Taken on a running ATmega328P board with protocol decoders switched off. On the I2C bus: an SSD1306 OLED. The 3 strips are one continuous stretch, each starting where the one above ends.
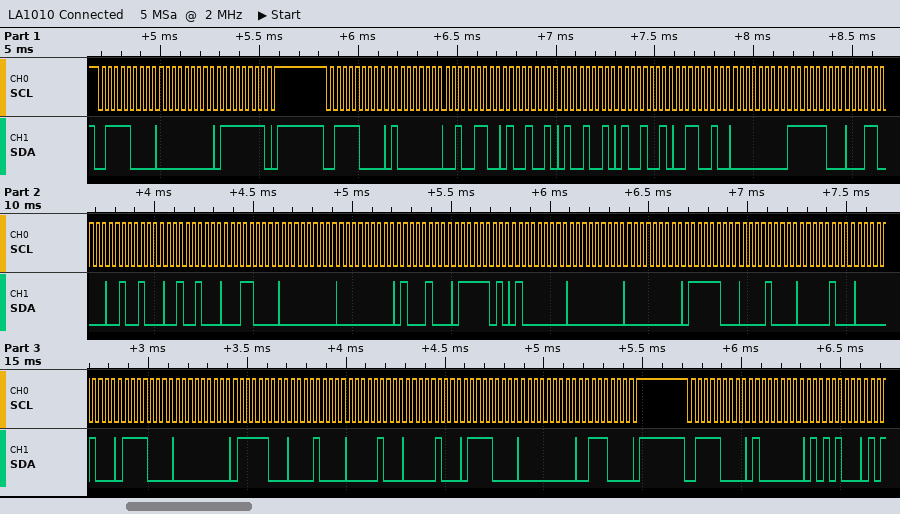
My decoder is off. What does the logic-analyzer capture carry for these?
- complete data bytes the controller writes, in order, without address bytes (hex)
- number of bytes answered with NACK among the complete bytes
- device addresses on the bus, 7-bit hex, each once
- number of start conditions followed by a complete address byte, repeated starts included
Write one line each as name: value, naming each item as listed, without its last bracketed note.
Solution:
complete data bytes the controller writes, in order, without address bytes: 00 7F 40 26 49 49 49 32 00 FC 18 24 24 18 00 00 44 7D 40 00 00 7C 08 04 04 78 00 7C 08 04 04 78 00 38 40 54
number of bytes answered with NACK among the complete bytes: 0
device addresses on the bus, 7-bit hex, each once: 0x3C
number of start conditions followed by a complete address byte, repeated starts included: 3
